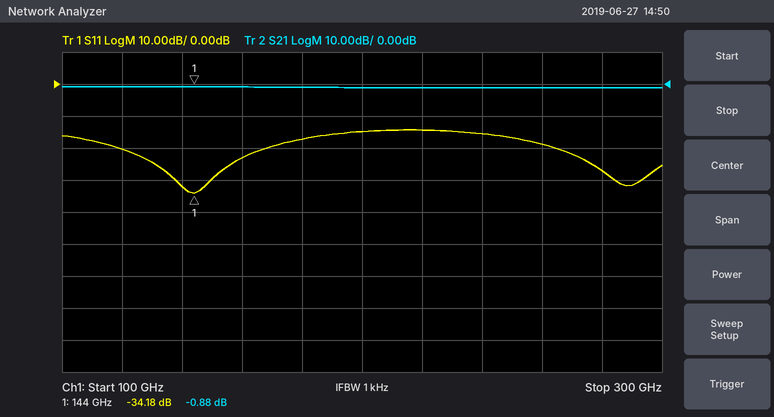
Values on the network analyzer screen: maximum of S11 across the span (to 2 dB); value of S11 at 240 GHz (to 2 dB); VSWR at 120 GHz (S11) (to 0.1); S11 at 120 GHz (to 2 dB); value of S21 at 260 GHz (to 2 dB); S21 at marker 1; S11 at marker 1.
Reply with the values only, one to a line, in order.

-14 dB
-16 dB
1.2
-20 dB
-2 dB
-0.88 dB
-34.18 dB
